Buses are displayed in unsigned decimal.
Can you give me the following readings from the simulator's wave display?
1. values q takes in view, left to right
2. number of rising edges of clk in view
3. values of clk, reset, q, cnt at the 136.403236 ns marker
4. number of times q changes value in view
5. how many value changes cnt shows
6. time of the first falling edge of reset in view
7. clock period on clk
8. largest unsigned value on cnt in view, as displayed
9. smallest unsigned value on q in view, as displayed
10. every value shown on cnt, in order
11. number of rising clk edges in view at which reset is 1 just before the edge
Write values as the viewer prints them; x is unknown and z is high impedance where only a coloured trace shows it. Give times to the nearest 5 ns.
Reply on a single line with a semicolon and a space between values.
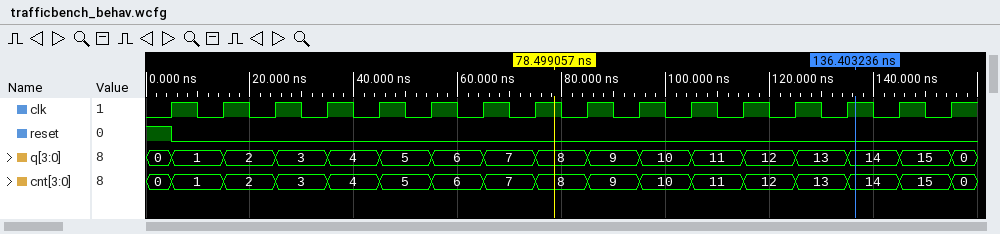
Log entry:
0, 1, 2, 3, 4, 5, 6, 7, 8, 9, 10, 11, 12, 13, 14, 15, 0; 16; clk=1, reset=0, q=14, cnt=14; 16; 16; 5 ns; 10 ns; 15; 0; 0, 1, 2, 3, 4, 5, 6, 7, 8, 9, 10, 11, 12, 13, 14, 15, 0; 1
